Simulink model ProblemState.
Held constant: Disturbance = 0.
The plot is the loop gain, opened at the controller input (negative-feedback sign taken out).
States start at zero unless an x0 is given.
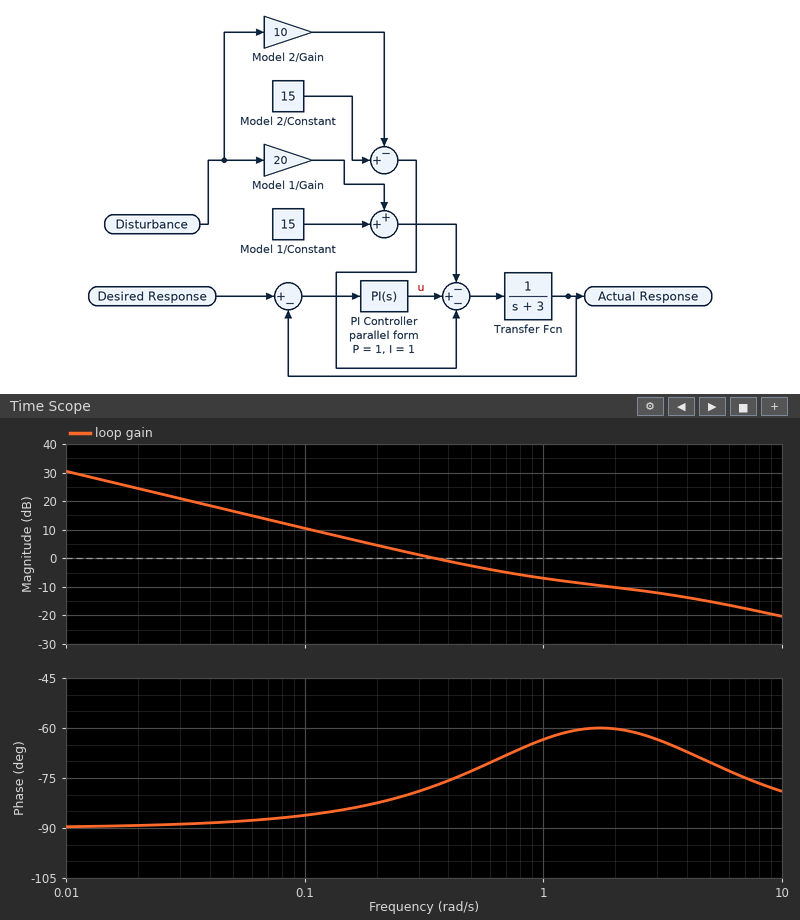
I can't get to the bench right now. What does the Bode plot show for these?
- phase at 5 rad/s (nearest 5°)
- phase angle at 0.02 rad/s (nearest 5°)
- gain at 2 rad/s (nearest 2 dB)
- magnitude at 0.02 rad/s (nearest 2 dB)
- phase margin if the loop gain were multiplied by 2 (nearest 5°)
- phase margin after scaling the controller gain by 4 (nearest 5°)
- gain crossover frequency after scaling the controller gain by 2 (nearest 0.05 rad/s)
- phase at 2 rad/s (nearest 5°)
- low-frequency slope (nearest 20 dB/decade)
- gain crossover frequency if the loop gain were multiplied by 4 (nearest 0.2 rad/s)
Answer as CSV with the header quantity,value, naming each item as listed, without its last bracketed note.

quantity,value
phase at 5 rad/s,-70°
phase angle at 0.02 rad/s,-90°
gain at 2 rad/s,-10 dB
magnitude at 0.02 rad/s,24 dB
phase margin if the loop gain were multiplied by 2,115°
phase margin after scaling the controller gain by 4,115°
gain crossover frequency after scaling the controller gain by 2,0.85 rad/s
phase at 2 rad/s,-60°
low-frequency slope,-20 dB/decade
gain crossover frequency if the loop gain were multiplied by 4,3.0 rad/s
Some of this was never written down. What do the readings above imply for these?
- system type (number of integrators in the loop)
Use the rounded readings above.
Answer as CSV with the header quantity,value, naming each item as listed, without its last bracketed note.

quantity,value
system type,1
